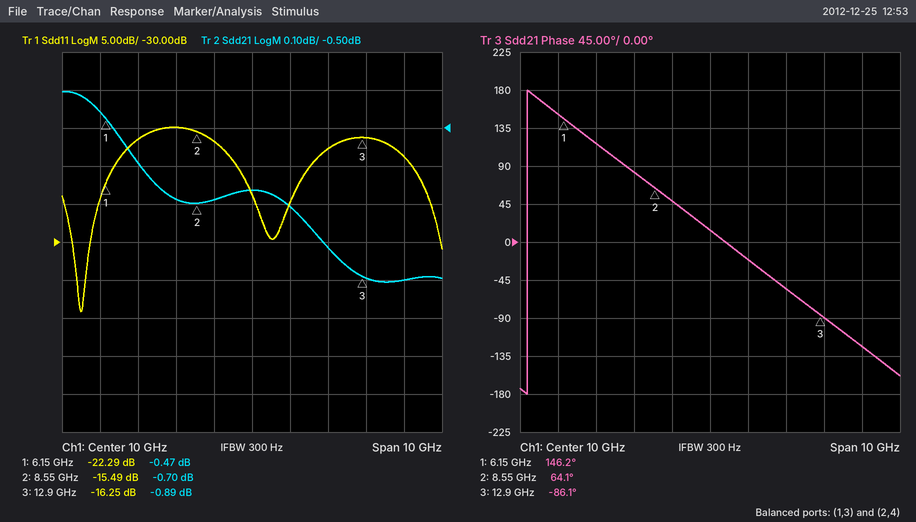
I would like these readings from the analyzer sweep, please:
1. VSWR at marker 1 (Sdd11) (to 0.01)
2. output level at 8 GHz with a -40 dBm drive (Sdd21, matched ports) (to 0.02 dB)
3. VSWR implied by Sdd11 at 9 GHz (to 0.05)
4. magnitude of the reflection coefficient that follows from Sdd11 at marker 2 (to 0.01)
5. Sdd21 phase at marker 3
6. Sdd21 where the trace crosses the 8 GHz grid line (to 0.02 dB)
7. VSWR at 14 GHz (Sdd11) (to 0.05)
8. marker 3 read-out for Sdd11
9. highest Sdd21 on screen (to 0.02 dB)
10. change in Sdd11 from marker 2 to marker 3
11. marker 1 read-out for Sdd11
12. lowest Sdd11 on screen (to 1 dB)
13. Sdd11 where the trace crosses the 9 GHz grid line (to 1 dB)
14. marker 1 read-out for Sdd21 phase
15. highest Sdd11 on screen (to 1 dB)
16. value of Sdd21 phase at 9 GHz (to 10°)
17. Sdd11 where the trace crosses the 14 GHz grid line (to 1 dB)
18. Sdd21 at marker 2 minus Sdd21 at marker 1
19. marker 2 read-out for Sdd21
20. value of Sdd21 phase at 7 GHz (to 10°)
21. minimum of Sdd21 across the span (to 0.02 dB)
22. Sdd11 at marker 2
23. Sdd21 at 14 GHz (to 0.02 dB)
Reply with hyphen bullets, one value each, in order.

- 1.17
- -40.68 dBm
- 1.35
- 0.17
- -86.1°
- -0.68 dB
- 1.25
- -16.25 dB
- -0.40 dB
- -0.76 dB
- -22.29 dB
- -39 dB
- -17 dB
- 146.2°
- -15 dB
- 50°
- -19 dB
- -0.23 dB
- -0.70 dB
- 120°
- -0.90 dB
- -15.49 dB
- -0.90 dB
